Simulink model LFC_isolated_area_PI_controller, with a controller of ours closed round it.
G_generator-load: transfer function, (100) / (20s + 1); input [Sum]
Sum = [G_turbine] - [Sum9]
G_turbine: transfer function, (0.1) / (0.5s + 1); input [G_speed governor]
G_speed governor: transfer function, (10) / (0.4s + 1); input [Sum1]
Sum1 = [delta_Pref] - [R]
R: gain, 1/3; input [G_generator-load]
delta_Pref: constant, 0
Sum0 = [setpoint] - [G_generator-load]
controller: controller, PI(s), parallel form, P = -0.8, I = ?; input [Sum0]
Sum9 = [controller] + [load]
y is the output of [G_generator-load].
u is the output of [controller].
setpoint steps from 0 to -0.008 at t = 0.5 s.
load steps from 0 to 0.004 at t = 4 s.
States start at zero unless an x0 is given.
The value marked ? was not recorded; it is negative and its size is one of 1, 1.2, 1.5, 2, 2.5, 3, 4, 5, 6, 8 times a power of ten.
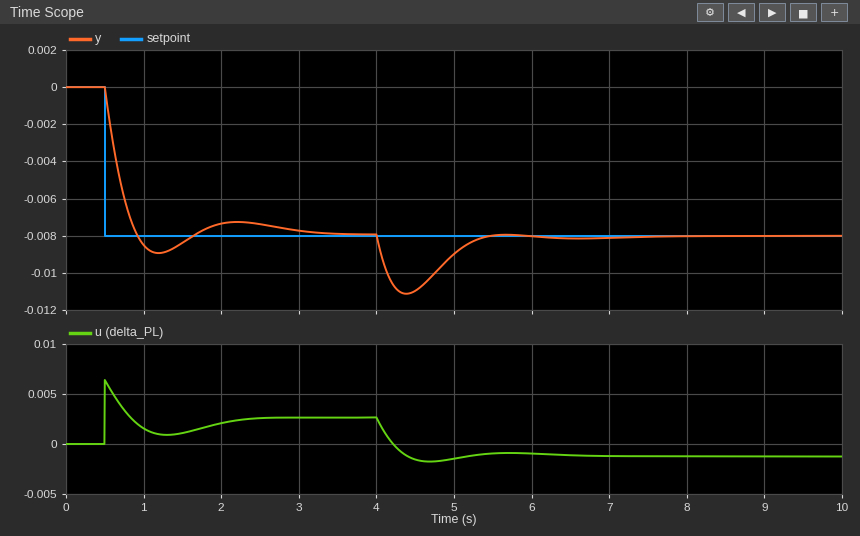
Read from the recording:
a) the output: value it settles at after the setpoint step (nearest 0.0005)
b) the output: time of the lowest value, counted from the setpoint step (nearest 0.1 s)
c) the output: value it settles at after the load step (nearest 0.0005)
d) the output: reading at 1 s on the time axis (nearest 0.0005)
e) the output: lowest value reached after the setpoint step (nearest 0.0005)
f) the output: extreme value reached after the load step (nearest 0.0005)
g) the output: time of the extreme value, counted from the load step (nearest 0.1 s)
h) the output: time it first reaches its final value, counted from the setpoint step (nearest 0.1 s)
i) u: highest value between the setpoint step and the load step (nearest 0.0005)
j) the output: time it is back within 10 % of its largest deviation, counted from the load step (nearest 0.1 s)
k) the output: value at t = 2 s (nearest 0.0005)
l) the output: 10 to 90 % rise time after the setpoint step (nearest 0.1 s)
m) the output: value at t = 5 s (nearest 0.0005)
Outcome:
-0.0080
0.7 s
-0.0080
-0.0085
-0.0090
-0.0110
0.4 s
0.4 s
0.0065
1.2 s
-0.0075
0.3 s
-0.0090
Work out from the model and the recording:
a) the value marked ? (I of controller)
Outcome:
-1.5
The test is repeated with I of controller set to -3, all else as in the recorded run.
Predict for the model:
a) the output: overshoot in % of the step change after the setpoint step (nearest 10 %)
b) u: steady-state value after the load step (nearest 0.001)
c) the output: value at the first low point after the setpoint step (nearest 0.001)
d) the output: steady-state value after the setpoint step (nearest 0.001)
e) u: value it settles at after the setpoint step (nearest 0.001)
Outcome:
20 %
-0.001
-0.010
-0.008
0.003
